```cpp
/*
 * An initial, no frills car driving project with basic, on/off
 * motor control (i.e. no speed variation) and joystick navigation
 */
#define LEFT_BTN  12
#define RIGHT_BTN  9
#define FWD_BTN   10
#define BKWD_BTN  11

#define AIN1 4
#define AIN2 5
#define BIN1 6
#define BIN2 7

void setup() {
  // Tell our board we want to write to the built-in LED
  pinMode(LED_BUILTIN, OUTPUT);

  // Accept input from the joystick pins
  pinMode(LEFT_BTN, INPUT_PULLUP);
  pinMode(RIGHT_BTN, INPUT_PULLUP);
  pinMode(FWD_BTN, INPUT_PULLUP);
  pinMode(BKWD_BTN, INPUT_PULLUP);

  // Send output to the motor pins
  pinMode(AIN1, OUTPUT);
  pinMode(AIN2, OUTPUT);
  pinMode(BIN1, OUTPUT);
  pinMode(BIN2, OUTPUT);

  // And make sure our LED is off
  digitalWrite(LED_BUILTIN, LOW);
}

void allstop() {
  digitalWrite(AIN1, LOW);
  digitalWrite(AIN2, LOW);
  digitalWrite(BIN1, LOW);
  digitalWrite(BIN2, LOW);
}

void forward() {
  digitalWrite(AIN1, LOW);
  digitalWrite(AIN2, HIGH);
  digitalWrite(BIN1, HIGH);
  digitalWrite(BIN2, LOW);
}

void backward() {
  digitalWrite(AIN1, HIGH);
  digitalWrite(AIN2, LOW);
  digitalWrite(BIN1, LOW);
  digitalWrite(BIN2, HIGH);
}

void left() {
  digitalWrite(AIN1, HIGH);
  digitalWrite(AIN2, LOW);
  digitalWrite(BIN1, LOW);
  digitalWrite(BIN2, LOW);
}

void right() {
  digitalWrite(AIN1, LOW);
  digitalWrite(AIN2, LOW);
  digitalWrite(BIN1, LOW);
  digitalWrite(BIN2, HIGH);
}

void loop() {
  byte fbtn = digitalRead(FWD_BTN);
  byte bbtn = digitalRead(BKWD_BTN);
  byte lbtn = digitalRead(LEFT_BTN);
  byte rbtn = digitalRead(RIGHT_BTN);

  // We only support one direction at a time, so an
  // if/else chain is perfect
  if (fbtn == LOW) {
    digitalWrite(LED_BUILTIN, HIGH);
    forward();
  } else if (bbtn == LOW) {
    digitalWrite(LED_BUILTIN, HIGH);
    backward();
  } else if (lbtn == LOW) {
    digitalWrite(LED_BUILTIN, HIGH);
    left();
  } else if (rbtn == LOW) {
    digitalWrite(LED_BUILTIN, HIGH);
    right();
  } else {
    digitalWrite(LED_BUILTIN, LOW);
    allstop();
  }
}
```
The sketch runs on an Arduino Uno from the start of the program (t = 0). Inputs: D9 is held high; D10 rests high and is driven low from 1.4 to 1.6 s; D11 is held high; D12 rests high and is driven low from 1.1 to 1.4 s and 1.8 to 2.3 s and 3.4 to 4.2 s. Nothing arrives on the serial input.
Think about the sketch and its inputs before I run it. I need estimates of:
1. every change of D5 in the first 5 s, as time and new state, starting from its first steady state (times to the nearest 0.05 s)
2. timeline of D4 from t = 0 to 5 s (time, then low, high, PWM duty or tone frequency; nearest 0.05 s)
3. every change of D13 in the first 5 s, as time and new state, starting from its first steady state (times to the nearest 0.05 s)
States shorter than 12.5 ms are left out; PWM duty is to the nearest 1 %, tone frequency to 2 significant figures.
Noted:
0 s low; 1.4 s high; 1.6 s low
0 s low; 1.1 s high; 1.4 s low; 1.8 s high; 2.3 s low; 3.4 s high; 4.2 s low
0 s low; 1.1 s high; 1.6 s low; 1.8 s high; 2.3 s low; 3.4 s high; 4.2 s low
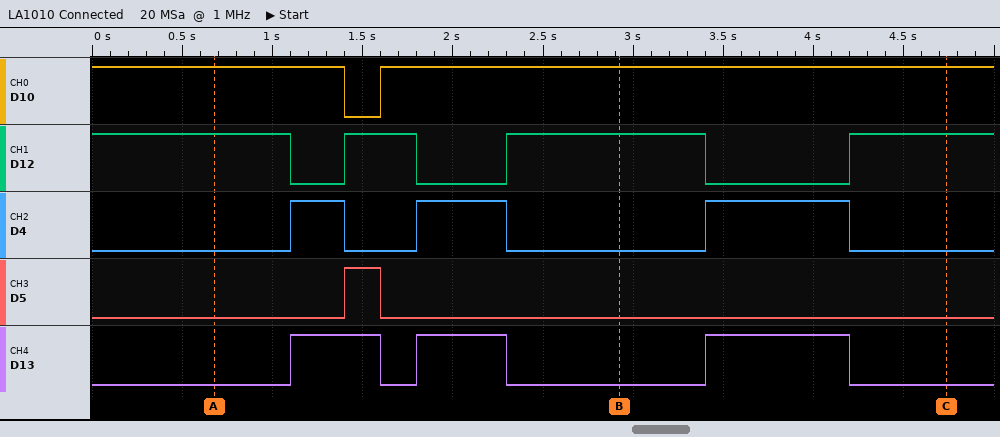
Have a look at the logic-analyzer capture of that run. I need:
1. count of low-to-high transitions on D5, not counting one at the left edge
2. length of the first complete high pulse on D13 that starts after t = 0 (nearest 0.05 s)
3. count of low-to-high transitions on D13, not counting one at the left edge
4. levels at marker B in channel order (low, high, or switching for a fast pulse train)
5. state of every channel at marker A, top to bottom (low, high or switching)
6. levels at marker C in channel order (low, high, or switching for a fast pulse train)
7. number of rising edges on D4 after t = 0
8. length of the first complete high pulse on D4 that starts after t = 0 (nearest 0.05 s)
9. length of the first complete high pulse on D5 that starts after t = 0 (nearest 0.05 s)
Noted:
1
0.50 s
3
D10 high, D12 high, D4 low, D5 low, D13 low
D10 high, D12 high, D4 low, D5 low, D13 low
D10 high, D12 high, D4 low, D5 low, D13 low
3
0.30 s
0.20 s
